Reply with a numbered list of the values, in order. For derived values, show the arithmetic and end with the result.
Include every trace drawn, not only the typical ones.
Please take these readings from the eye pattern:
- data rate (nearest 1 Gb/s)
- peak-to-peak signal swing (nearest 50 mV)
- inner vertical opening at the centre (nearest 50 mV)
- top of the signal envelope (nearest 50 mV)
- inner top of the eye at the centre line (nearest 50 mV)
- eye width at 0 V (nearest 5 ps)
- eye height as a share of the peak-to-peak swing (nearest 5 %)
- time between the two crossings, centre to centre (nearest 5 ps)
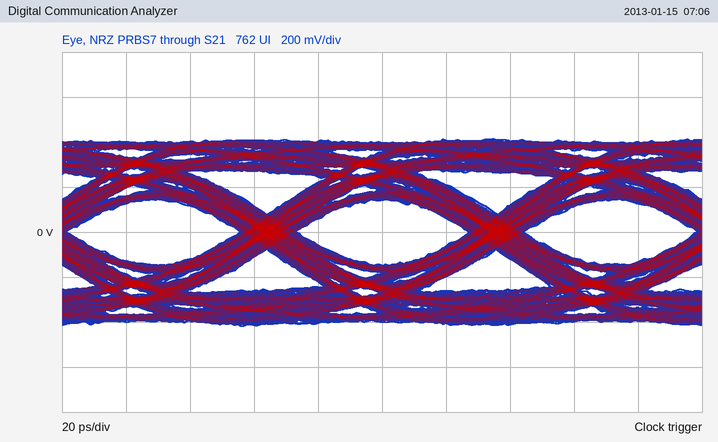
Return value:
1. 14 Gb/s
2. 850 mV
3. 300 mV
4. 400 mV
5. 150 mV
6. 55 ps
7. 300 mV / 850 mV ≈ 35 %
8. 70 ps
